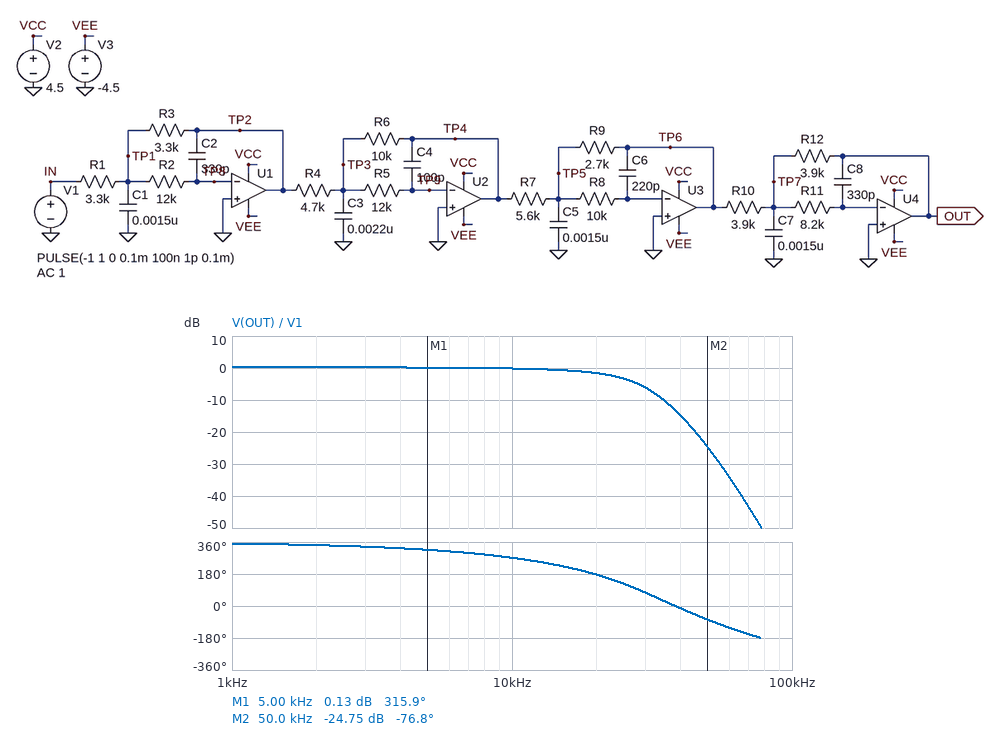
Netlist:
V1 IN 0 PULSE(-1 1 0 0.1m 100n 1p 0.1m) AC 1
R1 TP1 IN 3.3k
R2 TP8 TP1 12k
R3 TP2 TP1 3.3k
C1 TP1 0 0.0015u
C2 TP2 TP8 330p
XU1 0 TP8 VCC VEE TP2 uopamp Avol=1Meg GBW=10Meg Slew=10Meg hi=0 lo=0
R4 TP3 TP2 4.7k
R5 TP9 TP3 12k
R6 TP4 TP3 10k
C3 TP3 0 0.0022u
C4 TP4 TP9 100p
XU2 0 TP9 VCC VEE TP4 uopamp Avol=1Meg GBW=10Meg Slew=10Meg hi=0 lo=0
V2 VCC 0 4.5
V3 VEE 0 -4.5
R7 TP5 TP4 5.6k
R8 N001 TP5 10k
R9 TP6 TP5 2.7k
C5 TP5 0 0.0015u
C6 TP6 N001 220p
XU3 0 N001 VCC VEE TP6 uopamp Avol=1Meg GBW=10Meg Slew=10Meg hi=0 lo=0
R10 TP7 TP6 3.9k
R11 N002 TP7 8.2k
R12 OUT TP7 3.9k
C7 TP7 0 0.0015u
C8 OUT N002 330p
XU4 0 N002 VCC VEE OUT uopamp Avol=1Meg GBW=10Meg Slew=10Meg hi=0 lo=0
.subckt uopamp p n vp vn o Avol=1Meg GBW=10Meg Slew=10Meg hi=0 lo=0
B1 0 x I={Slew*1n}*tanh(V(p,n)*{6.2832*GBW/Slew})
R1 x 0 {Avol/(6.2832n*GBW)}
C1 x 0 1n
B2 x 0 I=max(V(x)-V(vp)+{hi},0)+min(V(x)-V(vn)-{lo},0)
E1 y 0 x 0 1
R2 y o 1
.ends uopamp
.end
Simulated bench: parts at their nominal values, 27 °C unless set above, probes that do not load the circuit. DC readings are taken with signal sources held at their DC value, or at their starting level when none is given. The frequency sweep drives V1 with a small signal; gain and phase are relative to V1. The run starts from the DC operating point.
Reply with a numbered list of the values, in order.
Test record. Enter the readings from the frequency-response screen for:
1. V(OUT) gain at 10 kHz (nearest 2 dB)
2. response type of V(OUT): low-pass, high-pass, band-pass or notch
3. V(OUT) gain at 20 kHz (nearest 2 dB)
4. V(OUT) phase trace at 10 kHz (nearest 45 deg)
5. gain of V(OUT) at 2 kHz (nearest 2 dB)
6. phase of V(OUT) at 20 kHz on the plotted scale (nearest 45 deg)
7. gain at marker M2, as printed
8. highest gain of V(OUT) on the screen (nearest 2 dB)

1. 0 dB
2. low-pass
3. -2 dB
4. 270 deg
5. 0 dB
6. 180 deg
7. -24.75 dB
8. 0 dB
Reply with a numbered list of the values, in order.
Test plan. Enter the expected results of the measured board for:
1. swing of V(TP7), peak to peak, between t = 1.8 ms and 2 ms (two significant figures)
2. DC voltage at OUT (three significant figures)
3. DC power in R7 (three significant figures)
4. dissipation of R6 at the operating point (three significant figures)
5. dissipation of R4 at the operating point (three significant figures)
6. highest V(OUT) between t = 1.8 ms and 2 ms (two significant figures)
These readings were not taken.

1. 370 mV
2. -1.03 V
3. 808 µW
4. 453 µW
5. 213 µW
6. 740 mV
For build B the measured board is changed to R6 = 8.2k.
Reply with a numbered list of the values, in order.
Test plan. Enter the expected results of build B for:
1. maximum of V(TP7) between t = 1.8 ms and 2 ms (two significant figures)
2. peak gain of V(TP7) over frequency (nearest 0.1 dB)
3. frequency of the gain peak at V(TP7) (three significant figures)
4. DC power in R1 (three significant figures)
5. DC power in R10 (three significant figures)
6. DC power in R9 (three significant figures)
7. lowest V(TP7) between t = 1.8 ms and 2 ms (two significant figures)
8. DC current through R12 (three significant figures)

1. 240 mV
2. -12.1 dB
3. 25.0 kHz
4. 303 µW
5. 181 µW
6. 262 µW
7. -74 mV
8. 216 µA
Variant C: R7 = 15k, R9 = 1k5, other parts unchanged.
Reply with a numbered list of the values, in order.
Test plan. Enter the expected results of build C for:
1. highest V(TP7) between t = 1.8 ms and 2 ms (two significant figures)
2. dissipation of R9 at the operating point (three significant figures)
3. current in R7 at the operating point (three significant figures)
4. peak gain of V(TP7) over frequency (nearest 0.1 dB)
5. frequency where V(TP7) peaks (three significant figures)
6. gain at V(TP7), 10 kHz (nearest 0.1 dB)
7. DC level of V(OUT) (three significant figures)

1. 58 mV
2. 30.2 µW
3. 142 µA
4. -24.2 dB
5. 23.6 kHz
6. -29.2 dB
7. -213 mV
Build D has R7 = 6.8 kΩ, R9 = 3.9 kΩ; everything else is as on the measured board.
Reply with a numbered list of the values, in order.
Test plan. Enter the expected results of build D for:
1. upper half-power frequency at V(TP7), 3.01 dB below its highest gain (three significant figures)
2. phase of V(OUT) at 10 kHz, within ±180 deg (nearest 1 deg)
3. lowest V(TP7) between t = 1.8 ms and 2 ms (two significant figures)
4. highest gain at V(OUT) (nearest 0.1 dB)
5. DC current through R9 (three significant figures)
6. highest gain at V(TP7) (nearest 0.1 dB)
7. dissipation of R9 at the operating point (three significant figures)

1. 33.0 kHz
2. -91 deg
3. -120 mV
4. 1.7 dB
5. 313 µA
6. -8.8 dB
7. 382 µW
